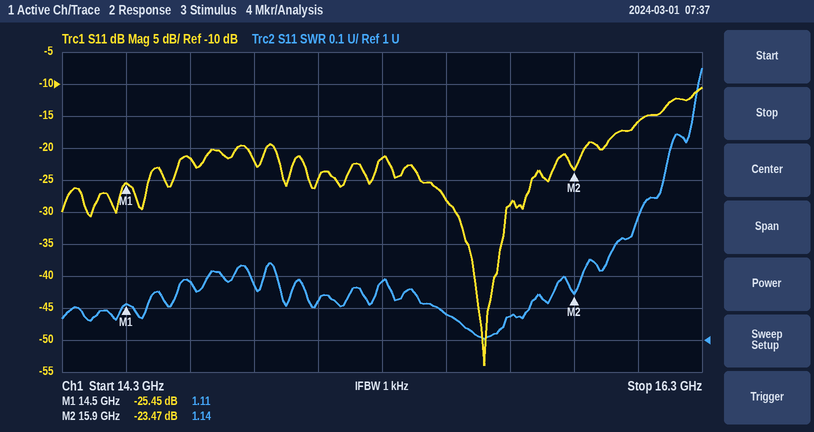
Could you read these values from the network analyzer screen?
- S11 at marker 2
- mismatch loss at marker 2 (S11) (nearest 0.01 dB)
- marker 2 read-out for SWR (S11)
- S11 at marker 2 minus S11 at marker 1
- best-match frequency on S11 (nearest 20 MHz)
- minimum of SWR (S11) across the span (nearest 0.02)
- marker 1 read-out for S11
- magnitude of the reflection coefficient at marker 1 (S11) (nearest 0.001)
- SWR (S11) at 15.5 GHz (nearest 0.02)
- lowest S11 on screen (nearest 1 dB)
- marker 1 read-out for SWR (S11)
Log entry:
-23.47 dB
0.02 dB
1.14
1.98 dB
15.62 GHz
1.00
-25.45 dB
0.053
1.08
-54 dB
1.11
